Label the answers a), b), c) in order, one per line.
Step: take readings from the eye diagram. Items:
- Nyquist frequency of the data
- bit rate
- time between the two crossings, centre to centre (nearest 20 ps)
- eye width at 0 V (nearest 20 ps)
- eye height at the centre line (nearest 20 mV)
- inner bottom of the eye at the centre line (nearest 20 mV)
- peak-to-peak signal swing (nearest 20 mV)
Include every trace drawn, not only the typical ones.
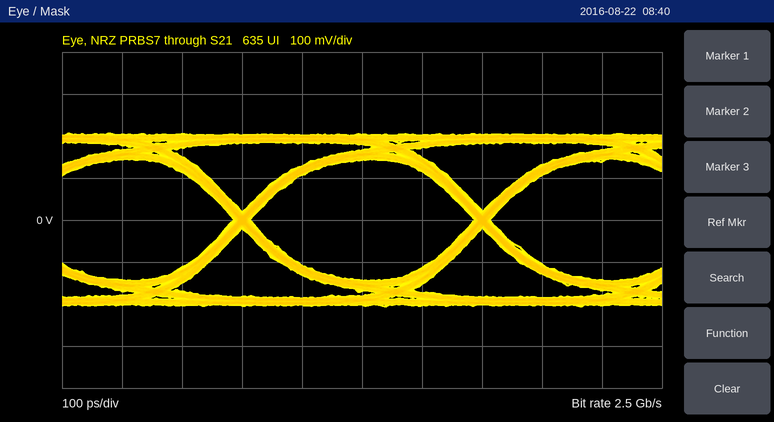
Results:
a) 1.25 GHz
b) 2.5 Gb/s
c) 400 ps
d) 380 ps
e) 280 mV
f) -140 mV
g) 420 mV
